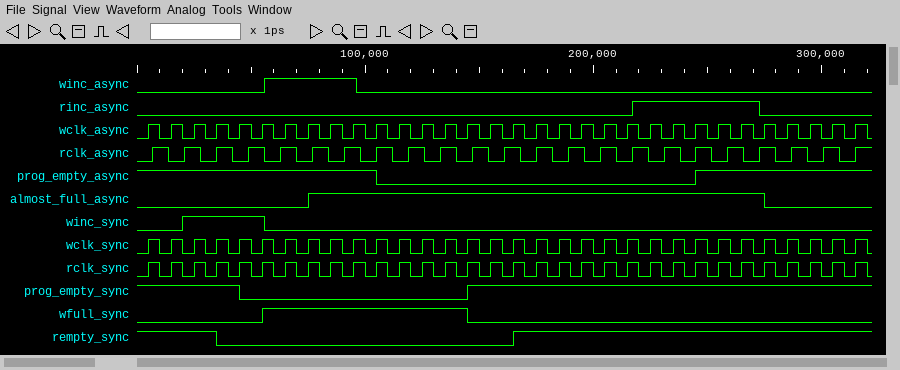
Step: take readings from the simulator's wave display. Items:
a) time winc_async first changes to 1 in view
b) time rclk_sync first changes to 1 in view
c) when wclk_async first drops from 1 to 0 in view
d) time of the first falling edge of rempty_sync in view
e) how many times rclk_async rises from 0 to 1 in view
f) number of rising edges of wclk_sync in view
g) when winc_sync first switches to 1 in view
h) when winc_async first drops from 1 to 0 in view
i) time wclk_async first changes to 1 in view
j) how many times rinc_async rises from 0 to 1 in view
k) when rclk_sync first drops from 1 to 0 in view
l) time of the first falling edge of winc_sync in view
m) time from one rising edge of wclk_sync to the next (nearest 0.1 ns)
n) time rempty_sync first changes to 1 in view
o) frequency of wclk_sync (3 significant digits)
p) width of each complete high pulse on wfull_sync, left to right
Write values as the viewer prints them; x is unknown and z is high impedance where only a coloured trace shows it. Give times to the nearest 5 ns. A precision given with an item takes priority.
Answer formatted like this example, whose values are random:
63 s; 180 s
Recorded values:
55 ns; 5 ns; 10 ns; 35 ns; 23; 32; 20 ns; 95 ns; 5 ns; 1; 10 ns; 55 ns; 10 ns; 165 ns; 100 MHz; 90 ns
